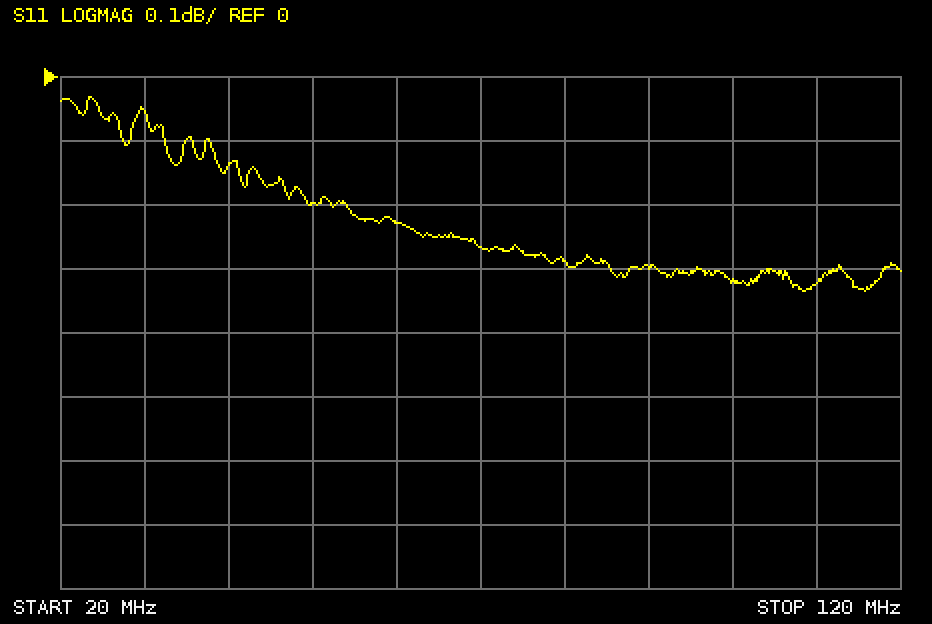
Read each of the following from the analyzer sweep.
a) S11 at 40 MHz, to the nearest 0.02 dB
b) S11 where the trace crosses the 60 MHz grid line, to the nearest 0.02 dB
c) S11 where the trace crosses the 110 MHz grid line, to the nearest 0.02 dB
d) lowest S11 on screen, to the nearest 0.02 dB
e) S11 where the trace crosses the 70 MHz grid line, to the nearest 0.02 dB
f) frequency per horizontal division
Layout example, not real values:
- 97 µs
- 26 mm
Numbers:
- -0.14 dB
- -0.22 dB
- -0.32 dB
- -0.34 dB
- -0.26 dB
- 10 MHz
